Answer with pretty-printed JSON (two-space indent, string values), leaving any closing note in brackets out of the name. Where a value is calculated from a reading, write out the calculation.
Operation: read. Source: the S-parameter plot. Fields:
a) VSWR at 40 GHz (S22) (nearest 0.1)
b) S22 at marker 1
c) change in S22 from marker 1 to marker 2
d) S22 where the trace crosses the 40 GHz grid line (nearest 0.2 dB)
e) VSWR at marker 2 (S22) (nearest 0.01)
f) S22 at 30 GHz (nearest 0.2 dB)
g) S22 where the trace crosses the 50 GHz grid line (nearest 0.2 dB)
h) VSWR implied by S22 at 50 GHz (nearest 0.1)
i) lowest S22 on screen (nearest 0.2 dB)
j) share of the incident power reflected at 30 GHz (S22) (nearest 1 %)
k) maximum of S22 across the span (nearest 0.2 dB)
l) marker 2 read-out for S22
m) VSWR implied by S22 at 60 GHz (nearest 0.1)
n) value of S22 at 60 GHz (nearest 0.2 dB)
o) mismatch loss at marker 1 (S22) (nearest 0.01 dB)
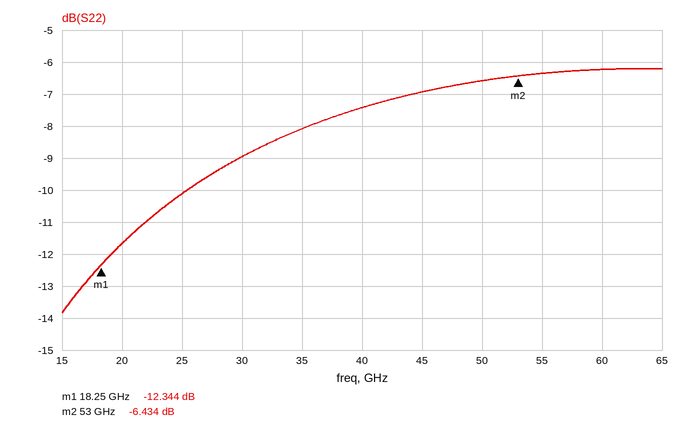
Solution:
{
  "VSWR at 40 GHz (S22)": "|Γ| = 10^(-7.4/20) = 0.4266; VSWR = (1 + 0.4266)/(1 − 0.4266) ≈ 2.5",
  "S22 at marker 1": "-12.344 dB",
  "change in S22 from marker 1 to marker 2": "-6.434 − (-12.344) = 5.910 dB",
  "S22 where the trace crosses the 40 GHz grid line": "-7.4 dB",
  "VSWR at marker 2 (S22)": "(1 + 0.4768)/(1 − 0.4768) ≈ 2.82",
  "S22 at 30 GHz": "-9.0 dB",
  "S22 where the trace crosses the 50 GHz grid line": "-6.6 dB",
  "VSWR implied by S22 at 50 GHz": "|Γ| = 10^(-6.6/20) = 0.4677; VSWR = (1 + 0.4677)/(1 − 0.4677) ≈ 2.8",
  "lowest S22 on screen": "-13.8 dB",
  "share of the incident power reflected at 30 GHz (S22)": "10^(-9/10) ≈ 13 %",
  "maximum of S22 across the span": "-6.2 dB",
  "marker 2 read-out for S22": "-6.434 dB",
  "VSWR implied by S22 at 60 GHz": "|Γ| = 10^(-6.2/20) = 0.4898; VSWR = (1 + 0.4898)/(1 − 0.4898) ≈ 2.9",
  "value of S22 at 60 GHz": "-6.2 dB",
  "mismatch loss at marker 1 (S22)": "−10 log10(1 − 10^(-12.344/10)) ≈ 0.26 dB"
}
